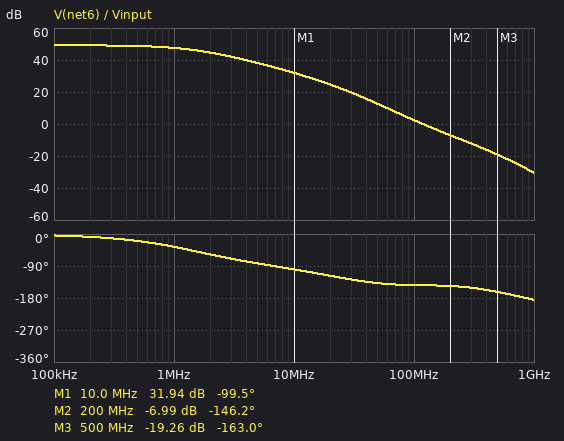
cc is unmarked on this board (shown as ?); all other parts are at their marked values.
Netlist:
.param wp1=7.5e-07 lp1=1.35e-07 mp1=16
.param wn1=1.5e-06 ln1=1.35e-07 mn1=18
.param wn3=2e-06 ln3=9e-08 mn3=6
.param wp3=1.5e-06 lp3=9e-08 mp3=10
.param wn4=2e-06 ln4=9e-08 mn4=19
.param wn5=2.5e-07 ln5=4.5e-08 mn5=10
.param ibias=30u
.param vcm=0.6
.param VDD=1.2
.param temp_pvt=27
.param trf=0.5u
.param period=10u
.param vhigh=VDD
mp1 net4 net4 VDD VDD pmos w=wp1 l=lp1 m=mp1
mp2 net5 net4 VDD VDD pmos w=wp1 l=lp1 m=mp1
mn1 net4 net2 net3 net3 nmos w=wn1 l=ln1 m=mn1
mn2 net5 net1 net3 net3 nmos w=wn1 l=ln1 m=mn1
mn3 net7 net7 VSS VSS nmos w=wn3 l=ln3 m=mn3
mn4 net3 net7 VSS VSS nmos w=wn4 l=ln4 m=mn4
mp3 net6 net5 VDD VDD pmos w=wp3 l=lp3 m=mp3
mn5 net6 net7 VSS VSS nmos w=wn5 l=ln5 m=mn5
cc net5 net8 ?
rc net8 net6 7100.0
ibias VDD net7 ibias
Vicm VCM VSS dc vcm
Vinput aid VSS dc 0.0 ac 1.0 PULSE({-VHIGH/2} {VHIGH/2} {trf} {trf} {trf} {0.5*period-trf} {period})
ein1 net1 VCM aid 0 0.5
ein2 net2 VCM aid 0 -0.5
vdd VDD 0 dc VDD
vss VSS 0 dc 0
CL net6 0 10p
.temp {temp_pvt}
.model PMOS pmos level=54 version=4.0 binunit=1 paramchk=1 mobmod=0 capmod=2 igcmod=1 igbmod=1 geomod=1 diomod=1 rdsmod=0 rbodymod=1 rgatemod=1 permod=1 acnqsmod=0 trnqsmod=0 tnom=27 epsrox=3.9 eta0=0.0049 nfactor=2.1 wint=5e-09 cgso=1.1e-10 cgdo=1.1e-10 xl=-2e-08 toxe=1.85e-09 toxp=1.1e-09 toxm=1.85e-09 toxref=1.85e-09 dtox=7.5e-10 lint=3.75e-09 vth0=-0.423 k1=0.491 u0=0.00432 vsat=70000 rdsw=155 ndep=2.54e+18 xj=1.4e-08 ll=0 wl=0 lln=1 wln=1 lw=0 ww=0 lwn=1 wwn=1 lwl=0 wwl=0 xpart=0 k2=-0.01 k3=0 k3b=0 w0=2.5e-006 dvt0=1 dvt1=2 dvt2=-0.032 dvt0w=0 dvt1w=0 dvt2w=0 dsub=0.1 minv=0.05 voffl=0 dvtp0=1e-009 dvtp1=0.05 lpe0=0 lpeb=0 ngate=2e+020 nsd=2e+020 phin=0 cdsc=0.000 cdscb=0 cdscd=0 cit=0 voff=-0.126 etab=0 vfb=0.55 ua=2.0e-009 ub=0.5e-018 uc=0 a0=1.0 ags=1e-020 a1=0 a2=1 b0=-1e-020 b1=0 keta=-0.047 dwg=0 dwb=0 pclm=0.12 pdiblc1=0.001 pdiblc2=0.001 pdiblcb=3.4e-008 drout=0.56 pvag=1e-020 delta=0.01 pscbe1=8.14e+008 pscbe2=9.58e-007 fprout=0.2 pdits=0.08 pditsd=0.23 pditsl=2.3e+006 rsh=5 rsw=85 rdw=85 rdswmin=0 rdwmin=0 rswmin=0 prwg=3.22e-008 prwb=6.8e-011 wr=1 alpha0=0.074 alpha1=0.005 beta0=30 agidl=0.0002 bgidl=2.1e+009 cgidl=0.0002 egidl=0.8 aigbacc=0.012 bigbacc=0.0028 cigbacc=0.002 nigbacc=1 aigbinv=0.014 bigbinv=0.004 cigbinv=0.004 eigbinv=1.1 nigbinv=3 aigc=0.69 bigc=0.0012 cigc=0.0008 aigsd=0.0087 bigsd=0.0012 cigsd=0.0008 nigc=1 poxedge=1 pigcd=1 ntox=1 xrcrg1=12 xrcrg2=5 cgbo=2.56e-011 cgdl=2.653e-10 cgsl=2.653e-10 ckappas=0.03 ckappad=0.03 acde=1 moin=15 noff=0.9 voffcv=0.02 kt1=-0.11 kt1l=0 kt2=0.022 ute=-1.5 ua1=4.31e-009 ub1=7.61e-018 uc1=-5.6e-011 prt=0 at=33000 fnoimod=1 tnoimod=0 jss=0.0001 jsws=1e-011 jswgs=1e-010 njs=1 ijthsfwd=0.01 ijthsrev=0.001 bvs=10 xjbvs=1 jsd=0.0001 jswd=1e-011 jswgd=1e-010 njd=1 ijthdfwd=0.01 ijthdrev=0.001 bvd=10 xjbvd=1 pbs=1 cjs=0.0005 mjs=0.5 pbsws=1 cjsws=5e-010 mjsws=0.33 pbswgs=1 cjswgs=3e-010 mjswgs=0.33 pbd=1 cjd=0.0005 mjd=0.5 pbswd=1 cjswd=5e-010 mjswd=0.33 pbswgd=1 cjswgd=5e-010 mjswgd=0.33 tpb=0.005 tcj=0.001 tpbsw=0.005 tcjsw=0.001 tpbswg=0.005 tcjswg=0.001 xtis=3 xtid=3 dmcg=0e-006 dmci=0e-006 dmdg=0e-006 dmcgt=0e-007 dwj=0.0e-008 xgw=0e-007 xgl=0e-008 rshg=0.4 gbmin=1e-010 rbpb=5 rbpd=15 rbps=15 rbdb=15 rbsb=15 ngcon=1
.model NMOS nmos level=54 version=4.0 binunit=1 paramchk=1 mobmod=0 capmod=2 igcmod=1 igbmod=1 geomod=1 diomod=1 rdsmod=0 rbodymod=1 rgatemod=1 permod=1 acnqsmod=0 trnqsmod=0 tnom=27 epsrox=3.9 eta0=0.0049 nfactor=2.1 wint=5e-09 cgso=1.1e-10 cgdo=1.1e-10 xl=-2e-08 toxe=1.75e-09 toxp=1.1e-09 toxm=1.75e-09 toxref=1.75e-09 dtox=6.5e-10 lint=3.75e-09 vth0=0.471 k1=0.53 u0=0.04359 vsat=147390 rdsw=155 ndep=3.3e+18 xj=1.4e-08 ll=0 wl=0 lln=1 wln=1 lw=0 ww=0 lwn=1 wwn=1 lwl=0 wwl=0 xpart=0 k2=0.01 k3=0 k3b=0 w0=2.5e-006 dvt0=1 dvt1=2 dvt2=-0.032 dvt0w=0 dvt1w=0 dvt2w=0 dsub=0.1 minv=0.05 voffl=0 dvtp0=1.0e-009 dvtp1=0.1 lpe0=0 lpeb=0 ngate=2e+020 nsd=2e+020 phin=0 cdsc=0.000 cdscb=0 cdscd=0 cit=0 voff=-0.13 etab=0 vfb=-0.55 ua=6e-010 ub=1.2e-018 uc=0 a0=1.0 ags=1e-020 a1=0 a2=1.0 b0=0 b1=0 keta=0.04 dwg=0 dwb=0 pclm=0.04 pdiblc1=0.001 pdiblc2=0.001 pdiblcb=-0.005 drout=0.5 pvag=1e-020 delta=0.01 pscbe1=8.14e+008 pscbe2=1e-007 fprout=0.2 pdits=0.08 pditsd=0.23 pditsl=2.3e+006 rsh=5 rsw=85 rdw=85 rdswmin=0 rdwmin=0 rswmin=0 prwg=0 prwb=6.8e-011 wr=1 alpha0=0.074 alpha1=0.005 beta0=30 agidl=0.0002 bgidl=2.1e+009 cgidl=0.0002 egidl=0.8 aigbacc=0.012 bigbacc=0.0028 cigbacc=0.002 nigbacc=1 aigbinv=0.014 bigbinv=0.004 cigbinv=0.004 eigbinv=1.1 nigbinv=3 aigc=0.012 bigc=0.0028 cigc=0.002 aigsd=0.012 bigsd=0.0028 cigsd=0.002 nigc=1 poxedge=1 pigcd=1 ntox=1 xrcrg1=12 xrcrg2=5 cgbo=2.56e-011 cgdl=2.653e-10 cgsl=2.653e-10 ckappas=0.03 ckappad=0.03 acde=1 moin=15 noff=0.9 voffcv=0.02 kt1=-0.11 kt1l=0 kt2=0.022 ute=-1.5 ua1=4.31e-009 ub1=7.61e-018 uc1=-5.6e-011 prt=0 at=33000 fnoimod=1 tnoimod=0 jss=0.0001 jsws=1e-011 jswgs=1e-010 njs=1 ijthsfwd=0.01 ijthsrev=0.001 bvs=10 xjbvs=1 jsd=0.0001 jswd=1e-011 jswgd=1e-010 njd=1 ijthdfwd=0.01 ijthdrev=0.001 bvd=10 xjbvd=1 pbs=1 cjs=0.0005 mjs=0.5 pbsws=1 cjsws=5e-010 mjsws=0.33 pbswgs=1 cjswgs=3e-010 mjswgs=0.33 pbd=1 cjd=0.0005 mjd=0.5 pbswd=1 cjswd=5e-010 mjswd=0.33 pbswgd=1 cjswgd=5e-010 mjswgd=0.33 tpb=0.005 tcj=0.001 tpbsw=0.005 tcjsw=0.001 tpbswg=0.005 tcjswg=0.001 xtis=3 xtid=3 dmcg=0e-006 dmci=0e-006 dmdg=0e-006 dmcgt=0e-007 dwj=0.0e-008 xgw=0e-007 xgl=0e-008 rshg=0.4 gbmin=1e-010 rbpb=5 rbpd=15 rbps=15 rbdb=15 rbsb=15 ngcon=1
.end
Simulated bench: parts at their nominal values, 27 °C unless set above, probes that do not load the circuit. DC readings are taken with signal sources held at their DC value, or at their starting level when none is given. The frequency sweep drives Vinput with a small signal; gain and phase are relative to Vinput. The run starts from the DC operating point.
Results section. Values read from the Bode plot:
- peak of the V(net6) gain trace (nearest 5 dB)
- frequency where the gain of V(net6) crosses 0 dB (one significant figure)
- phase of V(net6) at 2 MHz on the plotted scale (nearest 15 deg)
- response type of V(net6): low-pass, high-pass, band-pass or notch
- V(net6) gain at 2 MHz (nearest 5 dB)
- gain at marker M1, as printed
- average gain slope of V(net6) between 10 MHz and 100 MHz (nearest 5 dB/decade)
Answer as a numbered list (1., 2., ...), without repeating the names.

1. 50 dB
2. 100 MHz
3. -60 deg
4. low-pass
5. 45 dB
6. 31.94 dB
7. -30 dB/decade
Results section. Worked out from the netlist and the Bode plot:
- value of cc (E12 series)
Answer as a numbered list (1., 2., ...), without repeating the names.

1. 180 fF
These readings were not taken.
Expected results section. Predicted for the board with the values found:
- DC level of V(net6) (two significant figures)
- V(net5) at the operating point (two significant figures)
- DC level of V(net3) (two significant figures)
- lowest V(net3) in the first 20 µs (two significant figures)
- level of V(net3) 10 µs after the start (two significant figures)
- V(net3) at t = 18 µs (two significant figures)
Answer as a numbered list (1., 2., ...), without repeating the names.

1. 580 mV
2. 660 mV
3. 210 mV
4. 5.9 mV
5. 470 mV
6. 470 mV
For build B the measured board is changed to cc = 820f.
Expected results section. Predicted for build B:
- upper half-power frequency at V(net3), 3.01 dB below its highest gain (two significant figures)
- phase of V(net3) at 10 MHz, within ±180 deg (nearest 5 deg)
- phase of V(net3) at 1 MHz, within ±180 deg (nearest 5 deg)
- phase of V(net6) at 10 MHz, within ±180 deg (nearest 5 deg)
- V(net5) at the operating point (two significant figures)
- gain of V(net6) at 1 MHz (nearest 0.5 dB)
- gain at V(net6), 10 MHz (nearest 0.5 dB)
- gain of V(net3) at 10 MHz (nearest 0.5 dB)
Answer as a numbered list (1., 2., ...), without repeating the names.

1. 430 kHz
2. 155 deg
3. 125 deg
4. -95 deg
5. 660 mV
6. 41.0 dB
7. 21.5 dB
8. -32.0 dB
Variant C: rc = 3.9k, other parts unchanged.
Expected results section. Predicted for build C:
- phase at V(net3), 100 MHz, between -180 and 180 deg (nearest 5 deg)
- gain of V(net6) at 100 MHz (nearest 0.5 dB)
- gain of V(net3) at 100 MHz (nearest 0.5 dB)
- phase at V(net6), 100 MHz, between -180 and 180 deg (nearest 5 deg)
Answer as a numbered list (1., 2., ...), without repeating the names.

1. 155 deg
2. 1.5 dB
3. -30.0 dB
4. -155 deg
